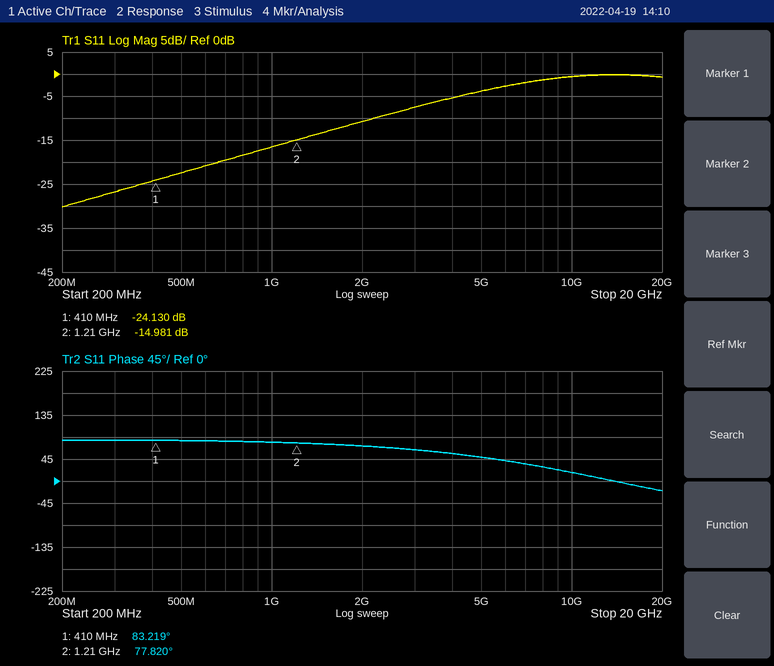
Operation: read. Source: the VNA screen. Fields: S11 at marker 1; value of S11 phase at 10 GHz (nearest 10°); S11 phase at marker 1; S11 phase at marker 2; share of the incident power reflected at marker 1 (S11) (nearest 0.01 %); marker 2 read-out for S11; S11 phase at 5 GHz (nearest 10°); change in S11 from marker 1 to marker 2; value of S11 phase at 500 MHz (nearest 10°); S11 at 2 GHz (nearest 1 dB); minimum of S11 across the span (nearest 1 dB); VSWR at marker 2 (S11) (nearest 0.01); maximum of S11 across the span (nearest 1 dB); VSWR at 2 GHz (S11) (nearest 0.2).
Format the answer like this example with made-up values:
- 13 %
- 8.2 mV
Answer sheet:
- -24.130 dB
- 20°
- 83.219°
- 77.820°
- 0.39 %
- -14.981 dB
- 50°
- 9.149 dB
- 80°
- -11 dB
- -30 dB
- 1.43
- 0 dB
- 1.8
